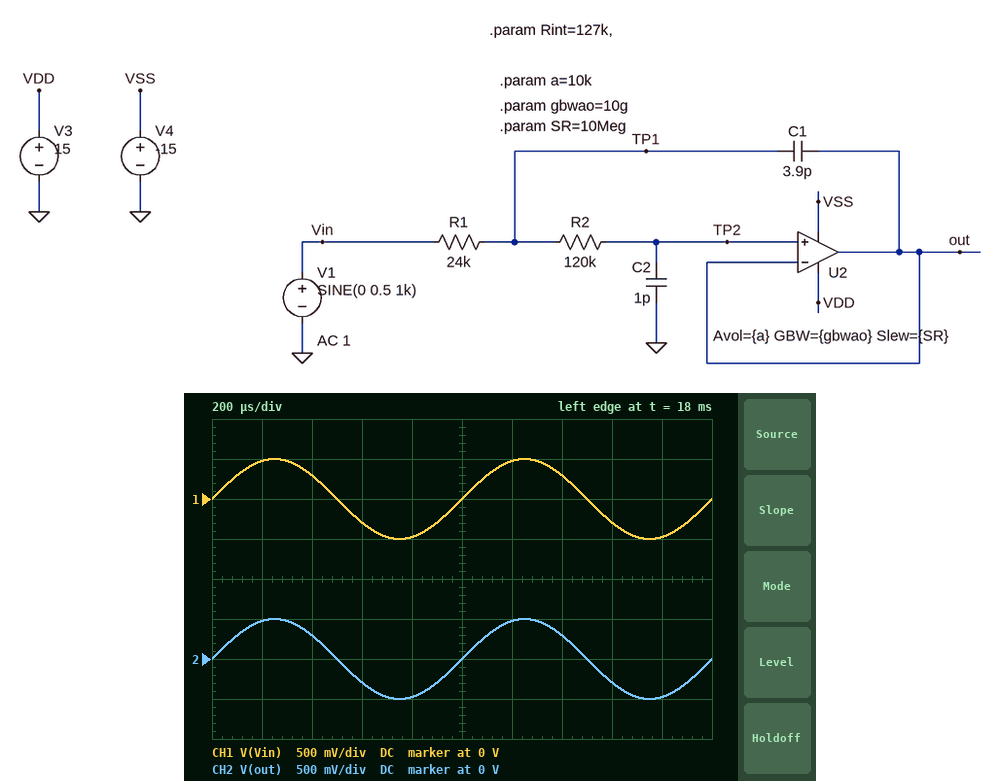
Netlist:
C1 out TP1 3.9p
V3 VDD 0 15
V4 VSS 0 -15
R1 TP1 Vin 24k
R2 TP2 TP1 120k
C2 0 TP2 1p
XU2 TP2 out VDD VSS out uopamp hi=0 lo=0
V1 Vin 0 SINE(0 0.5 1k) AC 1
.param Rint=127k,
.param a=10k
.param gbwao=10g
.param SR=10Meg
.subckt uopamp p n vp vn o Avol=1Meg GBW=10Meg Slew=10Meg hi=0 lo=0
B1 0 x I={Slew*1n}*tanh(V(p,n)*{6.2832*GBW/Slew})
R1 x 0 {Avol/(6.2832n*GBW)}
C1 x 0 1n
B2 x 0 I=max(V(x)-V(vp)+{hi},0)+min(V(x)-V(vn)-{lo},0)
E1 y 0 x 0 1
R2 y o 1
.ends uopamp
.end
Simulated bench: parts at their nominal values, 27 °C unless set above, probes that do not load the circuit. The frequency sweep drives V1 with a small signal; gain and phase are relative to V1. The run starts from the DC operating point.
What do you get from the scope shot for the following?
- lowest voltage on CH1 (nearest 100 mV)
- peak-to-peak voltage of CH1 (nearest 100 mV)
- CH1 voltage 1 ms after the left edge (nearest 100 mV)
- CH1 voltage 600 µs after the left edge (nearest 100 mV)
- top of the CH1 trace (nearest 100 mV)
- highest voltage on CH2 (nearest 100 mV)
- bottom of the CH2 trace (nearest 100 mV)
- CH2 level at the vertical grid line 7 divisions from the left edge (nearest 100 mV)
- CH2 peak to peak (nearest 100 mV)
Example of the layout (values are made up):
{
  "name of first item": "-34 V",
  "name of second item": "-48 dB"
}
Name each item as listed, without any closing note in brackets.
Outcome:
{
  "lowest voltage on CH1": "-500 mV",
  "peak-to-peak voltage of CH1": "1.0 V",
  "CH1 voltage 1 ms after the left edge": "0 V",
  "CH1 voltage 600 µs after the left edge": "-300 mV",
  "top of the CH1 trace": "500 mV",
  "highest voltage on CH2": "500 mV",
  "bottom of the CH2 trace": "-500 mV",
  "CH2 level at the vertical grid line 7 divisions from the left edge": "300 mV",
  "CH2 peak to peak": "1.0 V"
}
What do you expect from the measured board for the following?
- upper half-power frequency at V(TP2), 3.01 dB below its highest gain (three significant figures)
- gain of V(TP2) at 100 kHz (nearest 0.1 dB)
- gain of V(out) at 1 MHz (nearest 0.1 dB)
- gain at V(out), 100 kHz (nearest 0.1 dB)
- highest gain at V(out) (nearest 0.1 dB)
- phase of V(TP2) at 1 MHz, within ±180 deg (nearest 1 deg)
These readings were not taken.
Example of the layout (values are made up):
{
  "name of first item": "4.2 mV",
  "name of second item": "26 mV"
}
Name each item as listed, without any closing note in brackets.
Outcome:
{
  "upper half-power frequency at V(TP2), 3.01 dB below its highest gain": "1.51 MHz",
  "gain of V(TP2) at 100 kHz": "0 dB",
  "gain of V(out) at 1 MHz": "-0.4 dB",
  "gain at V(out), 100 kHz": "0 dB",
  "highest gain at V(out)": "0.1 dB",
  "phase of V(TP2) at 1 MHz, within ±180 deg": "-61 deg"
}
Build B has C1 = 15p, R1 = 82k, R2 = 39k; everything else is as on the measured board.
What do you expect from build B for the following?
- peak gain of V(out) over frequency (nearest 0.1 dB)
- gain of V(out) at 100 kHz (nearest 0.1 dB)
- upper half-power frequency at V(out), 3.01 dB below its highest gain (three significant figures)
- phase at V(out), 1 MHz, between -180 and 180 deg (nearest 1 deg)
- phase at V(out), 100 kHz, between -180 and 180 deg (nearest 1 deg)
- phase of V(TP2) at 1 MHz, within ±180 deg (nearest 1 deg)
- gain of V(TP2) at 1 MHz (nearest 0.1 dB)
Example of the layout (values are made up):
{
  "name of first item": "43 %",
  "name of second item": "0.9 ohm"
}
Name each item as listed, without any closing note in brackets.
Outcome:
{
  "peak gain of V(out) over frequency": "6.6 dB",
  "gain of V(out) at 100 kHz": "0.2 dB",
  "upper half-power frequency at V(out), 3.01 dB below its highest gain": "709 kHz",
  "phase at V(out), 1 MHz, between -180 and 180 deg": "-159 deg",
  "phase at V(out), 100 kHz, between -180 and 180 deg": "-5 deg",
  "phase of V(TP2) at 1 MHz, within ±180 deg": "-153 deg",
  "gain of V(TP2) at 1 MHz": "-5.4 dB"
}
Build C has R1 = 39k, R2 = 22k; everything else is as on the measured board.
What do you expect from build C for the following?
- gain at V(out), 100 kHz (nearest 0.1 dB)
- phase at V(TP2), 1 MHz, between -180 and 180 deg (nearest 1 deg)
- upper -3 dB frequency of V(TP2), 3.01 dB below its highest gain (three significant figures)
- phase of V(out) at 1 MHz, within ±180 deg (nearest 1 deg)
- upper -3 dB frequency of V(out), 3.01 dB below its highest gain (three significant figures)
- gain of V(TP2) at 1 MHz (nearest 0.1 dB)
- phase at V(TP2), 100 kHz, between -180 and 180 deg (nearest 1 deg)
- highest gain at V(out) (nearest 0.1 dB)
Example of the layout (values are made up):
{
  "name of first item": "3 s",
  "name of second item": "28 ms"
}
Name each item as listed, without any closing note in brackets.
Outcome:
{
  "gain at V(out), 100 kHz": "0 dB",
  "phase at V(TP2), 1 MHz, between -180 and 180 deg": "-27 deg",
  "upper -3 dB frequency of V(TP2), 3.01 dB below its highest gain": "2.42 MHz",
  "phase of V(out) at 1 MHz, within ±180 deg": "-33 deg",
  "upper -3 dB frequency of V(out), 3.01 dB below its highest gain": "2.40 MHz",
  "gain of V(TP2) at 1 MHz": "1.2 dB",
  "phase at V(TP2), 100 kHz, between -180 and 180 deg": "-2 deg",
  "highest gain at V(out)": "2.1 dB"
}
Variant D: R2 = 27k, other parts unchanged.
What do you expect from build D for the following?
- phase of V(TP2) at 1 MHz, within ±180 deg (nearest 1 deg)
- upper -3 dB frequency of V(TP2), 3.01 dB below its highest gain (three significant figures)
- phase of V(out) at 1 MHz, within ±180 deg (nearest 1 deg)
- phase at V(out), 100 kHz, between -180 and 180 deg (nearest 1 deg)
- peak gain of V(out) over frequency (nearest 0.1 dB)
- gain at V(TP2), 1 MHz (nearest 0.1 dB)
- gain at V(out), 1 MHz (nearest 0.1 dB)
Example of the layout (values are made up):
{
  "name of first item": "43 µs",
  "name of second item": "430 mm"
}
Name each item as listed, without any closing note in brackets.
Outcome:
{
  "phase of V(TP2) at 1 MHz, within ±180 deg": "-21 deg",
  "upper -3 dB frequency of V(TP2), 3.01 dB below its highest gain": "2.90 MHz",
  "phase of V(out) at 1 MHz, within ±180 deg": "-27 deg",
  "phase at V(out), 100 kHz, between -180 and 180 deg": "-2 deg",
  "peak gain of V(out) over frequency": "2.0 dB",
  "gain at V(TP2), 1 MHz": "0.9 dB",
  "gain at V(out), 1 MHz": "0.8 dB"
}
